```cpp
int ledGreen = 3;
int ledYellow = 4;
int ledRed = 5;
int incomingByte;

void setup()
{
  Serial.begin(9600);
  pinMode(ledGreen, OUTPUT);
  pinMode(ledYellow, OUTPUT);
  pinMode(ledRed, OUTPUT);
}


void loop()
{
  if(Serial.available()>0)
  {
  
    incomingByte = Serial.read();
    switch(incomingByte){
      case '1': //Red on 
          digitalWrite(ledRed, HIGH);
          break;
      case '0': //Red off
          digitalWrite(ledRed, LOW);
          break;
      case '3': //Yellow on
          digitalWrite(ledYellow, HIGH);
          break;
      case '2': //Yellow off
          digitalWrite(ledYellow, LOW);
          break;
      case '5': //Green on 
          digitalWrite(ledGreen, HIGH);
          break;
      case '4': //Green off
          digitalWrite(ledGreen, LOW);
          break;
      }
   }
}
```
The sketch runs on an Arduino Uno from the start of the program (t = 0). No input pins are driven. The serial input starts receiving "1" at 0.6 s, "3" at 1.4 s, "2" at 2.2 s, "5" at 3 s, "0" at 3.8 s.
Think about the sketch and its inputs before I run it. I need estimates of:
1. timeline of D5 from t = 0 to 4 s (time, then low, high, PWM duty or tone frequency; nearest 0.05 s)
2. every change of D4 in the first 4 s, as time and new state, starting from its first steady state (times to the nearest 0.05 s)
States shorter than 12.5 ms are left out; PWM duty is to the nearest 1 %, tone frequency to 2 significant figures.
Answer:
0 s low; 0.6 s high; 3.8 s low
0 s low; 1.4 s high; 2.2 s low
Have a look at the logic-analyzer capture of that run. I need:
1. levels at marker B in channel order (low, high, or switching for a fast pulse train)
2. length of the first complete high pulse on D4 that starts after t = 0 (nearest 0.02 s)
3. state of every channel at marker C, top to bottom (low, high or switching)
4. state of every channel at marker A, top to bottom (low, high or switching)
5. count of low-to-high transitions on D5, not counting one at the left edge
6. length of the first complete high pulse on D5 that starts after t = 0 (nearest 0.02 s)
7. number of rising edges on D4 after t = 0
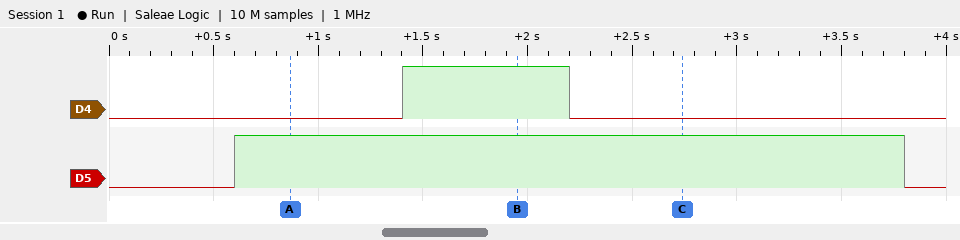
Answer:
D4 high, D5 high
0.80 s
D4 low, D5 high
D4 low, D5 high
1
3.20 s
1
